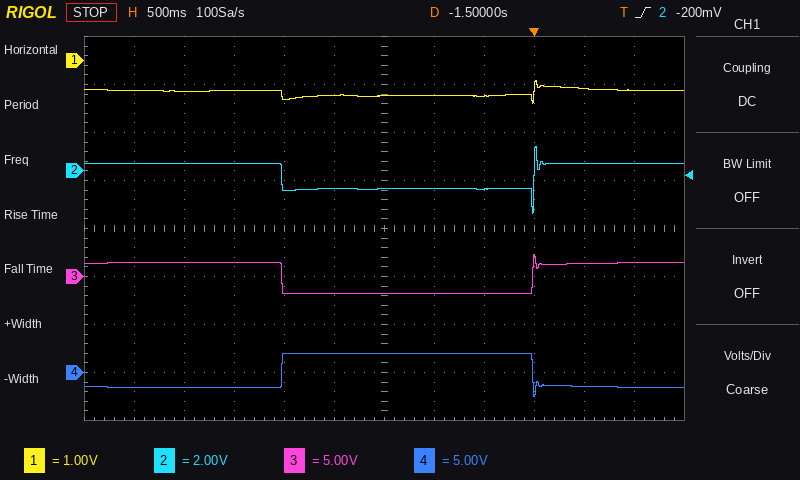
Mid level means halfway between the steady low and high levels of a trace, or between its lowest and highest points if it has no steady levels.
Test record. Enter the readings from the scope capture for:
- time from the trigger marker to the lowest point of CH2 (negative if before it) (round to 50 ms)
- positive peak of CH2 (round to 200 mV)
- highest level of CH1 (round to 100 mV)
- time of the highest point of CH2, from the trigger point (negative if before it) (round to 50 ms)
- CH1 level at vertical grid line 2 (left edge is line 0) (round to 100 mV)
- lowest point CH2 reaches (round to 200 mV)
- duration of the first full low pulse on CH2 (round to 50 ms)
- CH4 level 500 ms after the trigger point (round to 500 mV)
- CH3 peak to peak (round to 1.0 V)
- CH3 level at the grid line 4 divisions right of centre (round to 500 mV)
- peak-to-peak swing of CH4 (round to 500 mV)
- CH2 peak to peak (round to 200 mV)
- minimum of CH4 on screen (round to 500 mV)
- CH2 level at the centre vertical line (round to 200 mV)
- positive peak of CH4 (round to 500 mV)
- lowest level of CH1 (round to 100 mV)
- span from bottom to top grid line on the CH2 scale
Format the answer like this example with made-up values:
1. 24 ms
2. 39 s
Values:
1. 0 ms
2. 1.0 V
3. -400 mV
4. 0 ms
5. -600 mV
6. -1.8 V
7. 2.50 s
8. -1.5 V
9. 4.0 V
10. 1.5 V
11. 4.5 V
12. 2.8 V
13. -2.5 V
14. -800 mV
15. 2.0 V
16. -900 mV
17. 16 V
